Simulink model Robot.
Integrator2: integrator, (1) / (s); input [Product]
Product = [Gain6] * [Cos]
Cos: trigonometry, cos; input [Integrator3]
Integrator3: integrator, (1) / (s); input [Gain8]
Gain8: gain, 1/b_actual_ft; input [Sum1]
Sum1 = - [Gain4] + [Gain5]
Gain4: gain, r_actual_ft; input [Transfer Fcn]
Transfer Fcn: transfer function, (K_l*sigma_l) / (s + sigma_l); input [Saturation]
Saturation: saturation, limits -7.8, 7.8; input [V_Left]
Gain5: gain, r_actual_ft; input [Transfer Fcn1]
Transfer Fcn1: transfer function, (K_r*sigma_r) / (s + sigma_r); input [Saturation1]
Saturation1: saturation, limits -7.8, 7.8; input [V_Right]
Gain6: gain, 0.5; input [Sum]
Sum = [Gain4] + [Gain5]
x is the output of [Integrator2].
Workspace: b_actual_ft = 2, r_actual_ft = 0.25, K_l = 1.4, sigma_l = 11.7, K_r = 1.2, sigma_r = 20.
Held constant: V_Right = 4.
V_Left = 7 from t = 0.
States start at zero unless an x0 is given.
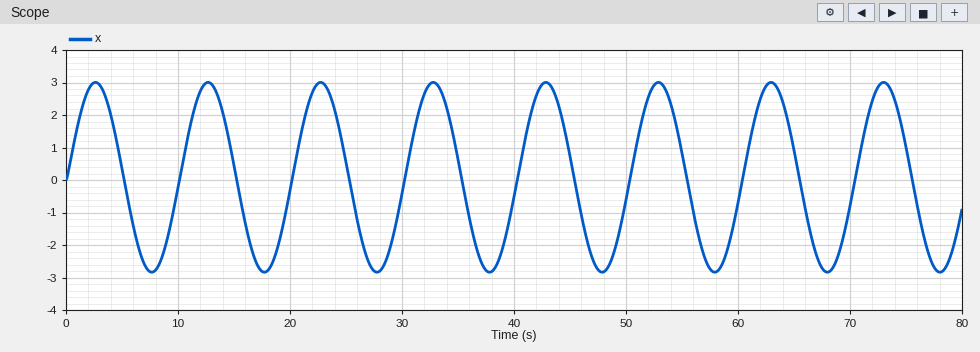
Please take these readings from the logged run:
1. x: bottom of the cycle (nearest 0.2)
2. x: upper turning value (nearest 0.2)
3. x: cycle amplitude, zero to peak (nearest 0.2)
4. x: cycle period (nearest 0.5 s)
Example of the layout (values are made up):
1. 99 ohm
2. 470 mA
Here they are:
1. -2.8
2. 3.0
3. 3.0
4. 10.0 s
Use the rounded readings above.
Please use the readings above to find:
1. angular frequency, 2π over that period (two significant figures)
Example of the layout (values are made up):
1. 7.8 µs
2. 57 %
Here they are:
1. 0.63 rad/s
